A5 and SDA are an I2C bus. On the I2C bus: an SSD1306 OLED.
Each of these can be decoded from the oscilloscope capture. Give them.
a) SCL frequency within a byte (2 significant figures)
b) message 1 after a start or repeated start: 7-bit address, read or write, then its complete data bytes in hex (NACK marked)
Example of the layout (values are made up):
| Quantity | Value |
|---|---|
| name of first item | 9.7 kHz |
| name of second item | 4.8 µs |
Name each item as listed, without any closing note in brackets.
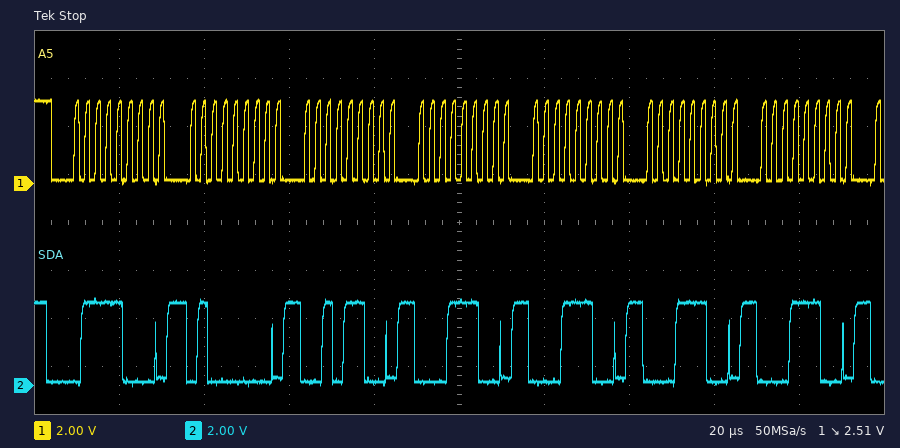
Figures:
| Quantity | Value |
|---|---|
| SCL frequency within a byte | 400 kHz |
| message 1 after a start or repeated start: 7-bit address, read or write, then its complete data bytes in hex | 0x3C write: 40 2C 1C 1C 1C 1C |
